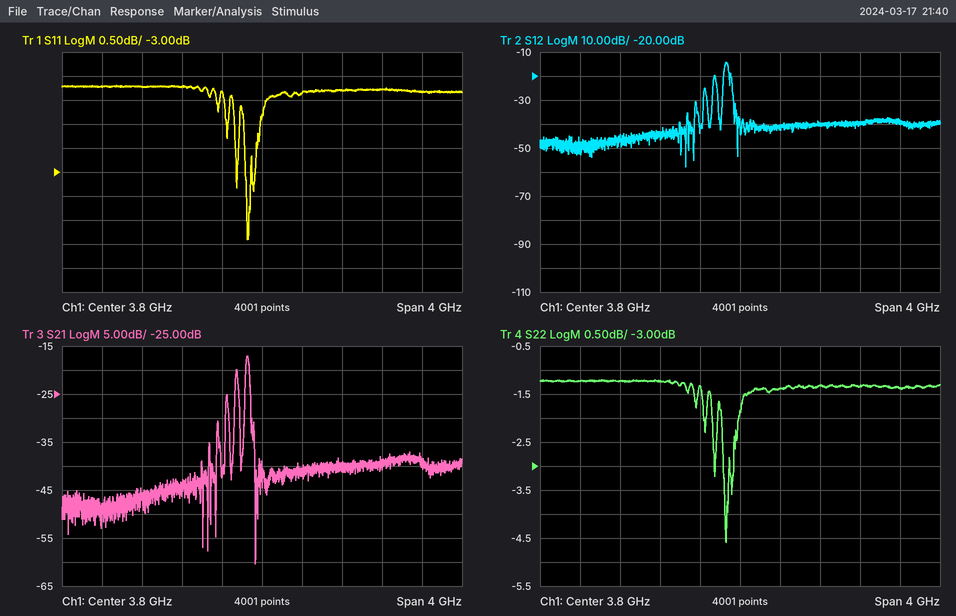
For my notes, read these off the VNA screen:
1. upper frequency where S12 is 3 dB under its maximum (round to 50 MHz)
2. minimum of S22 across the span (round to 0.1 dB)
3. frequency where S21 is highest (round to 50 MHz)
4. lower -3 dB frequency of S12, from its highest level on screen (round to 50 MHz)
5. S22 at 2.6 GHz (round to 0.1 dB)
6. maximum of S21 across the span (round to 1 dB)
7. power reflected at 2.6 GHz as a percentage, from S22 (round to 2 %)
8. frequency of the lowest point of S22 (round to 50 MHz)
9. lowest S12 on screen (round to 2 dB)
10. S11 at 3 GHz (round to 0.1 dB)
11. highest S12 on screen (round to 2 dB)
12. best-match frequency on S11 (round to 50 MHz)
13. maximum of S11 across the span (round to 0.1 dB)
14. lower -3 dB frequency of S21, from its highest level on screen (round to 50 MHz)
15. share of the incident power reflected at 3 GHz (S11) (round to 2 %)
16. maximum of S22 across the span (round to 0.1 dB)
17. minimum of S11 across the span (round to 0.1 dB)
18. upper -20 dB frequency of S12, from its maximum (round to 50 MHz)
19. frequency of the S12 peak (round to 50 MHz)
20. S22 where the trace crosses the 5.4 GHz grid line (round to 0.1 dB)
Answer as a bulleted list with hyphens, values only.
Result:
- 3.70 GHz
- -4.6 dB
- 3.65 GHz
- 3.65 GHz
- -1.2 dB
- -17 dB
- 76 %
- 3.65 GHz
- -58 dB
- -1.2 dB
- -14 dB
- 3.65 GHz
- -1.2 dB
- 3.65 GHz
- 76 %
- -1.2 dB
- -4.4 dB
- 3.75 GHz
- 3.65 GHz
- -1.4 dB
